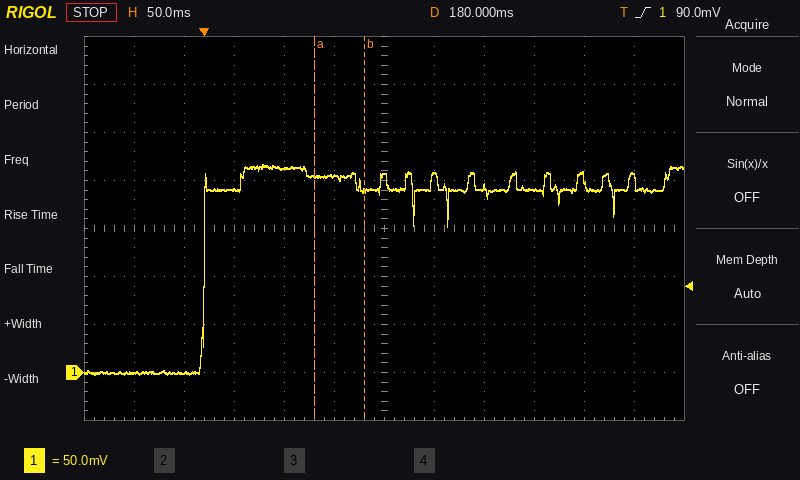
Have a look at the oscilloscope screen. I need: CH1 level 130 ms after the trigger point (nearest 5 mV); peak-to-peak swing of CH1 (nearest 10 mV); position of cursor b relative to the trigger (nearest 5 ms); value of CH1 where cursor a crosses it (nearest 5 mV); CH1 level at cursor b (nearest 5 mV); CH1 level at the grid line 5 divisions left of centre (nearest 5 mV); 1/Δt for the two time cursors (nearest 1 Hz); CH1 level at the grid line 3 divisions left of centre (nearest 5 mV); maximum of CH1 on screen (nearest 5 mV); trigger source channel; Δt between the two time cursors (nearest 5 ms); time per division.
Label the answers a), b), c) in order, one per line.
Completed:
a) 205 mV
b) 220 mV
c) +160 ms
d) 205 mV
e) 190 mV
f) 0 mV
g) 20 Hz
h) 190 mV
i) 215 mV
j) CH1
k) 50 ms
l) 50 ms
